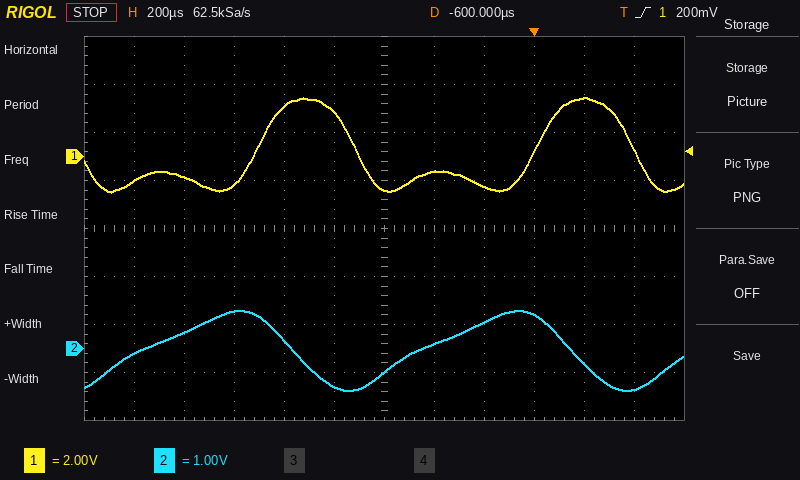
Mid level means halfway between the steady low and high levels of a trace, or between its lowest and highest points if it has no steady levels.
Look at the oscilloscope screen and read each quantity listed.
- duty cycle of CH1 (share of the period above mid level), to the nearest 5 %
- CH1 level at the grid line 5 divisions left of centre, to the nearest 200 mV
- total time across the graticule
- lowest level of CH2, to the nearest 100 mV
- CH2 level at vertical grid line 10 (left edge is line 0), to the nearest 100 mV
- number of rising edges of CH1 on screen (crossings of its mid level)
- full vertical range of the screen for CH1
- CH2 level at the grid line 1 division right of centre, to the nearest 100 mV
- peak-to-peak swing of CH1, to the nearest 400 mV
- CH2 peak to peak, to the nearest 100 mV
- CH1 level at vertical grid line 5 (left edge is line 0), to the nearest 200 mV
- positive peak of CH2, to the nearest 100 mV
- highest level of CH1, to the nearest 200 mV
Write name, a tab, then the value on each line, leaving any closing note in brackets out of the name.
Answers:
duty cycle of CH1 (share of the period above mid level), to the nearest 5 %	35 %
CH1 level at the grid line 5 divisions left of centre, to the nearest 200 mV	-1.0 V
total time across the graticule	2.4 ms
lowest level of CH2, to the nearest 100 mV	-900 mV
CH2 level at vertical grid line 10 (left edge is line 0), to the nearest 100 mV	-300 mV
number of rising edges of CH1 on screen	2
full vertical range of the screen for CH1	16 V
CH2 level at the grid line 1 division right of centre, to the nearest 100 mV	100 mV
peak-to-peak swing of CH1, to the nearest 400 mV	4.0 V
CH2 peak to peak, to the nearest 100 mV	1.7 V
CH1 level at vertical grid line 5 (left edge is line 0), to the nearest 200 mV	1.8 V
positive peak of CH2, to the nearest 100 mV	800 mV
highest level of CH1, to the nearest 200 mV	2.4 V
